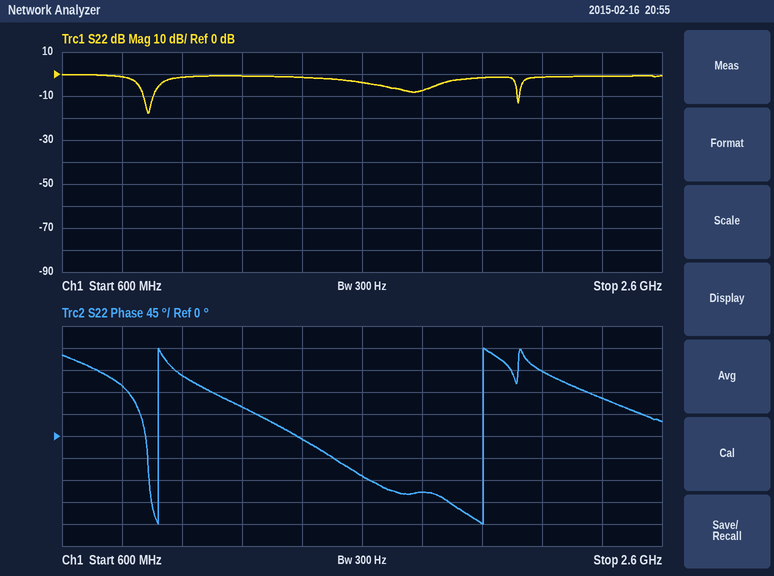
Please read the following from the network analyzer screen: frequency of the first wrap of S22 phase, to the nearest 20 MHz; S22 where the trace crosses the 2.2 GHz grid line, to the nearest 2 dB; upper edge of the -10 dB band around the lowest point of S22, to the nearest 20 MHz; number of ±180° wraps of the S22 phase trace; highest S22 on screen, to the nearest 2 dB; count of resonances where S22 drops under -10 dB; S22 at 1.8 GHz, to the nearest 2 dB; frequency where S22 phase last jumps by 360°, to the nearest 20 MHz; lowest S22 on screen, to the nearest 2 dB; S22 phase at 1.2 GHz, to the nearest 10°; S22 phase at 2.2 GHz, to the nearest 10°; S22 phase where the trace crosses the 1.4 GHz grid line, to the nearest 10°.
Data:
920 MHz
-2 dB
900 MHz
2
0 dB
2
-8 dB
2.00 GHz
-18 dB
60°
130°
-10°
